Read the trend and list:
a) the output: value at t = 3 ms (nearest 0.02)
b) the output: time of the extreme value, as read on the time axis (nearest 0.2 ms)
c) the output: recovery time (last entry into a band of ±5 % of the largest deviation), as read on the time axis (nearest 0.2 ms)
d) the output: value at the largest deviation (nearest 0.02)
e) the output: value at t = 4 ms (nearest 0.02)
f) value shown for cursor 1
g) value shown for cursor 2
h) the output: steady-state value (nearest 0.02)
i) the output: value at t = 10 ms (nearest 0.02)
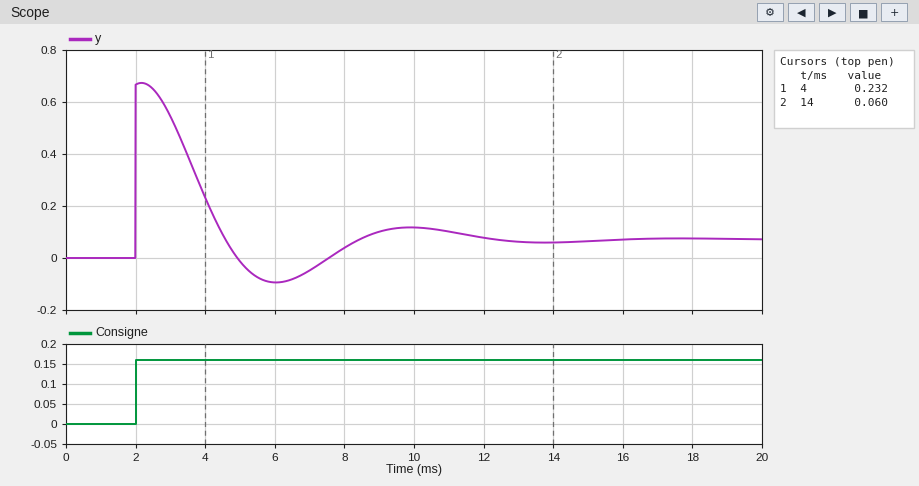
0.54
2.2 ms
10.8 ms
0.68
0.24
0.232
0.060
0.08
0.12
